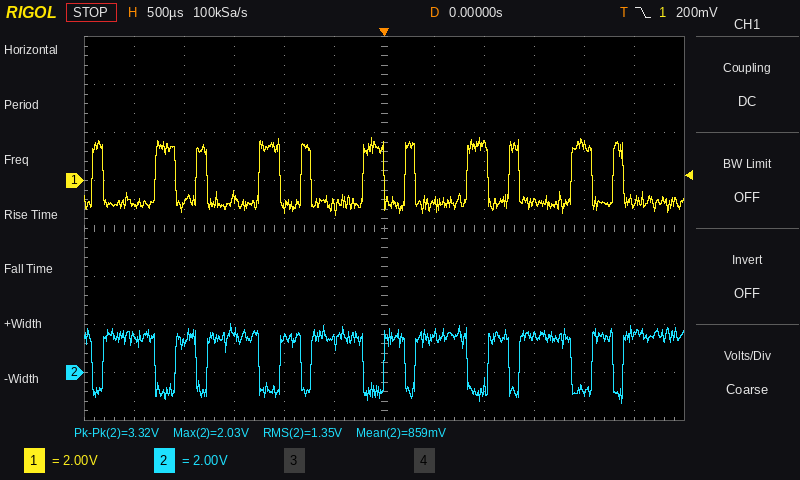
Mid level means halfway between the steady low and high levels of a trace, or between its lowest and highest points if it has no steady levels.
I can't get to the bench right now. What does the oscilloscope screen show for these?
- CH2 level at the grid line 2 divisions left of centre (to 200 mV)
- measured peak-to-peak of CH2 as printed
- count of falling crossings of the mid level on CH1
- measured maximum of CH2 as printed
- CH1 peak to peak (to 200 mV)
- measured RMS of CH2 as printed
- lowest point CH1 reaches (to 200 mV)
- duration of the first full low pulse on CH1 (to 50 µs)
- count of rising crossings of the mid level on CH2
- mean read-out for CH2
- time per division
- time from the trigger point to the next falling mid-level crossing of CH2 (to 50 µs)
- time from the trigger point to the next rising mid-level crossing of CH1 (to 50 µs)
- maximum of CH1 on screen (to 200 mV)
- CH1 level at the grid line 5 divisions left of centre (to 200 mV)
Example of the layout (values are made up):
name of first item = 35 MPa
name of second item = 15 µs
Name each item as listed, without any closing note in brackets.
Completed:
CH2 level at the grid line 2 divisions left of centre = 1.4 V
measured peak-to-peak of CH2 as printed = 3.32 V
count of falling crossings of the mid level on CH1 = 11
measured maximum of CH2 as printed = 2.03 V
CH1 peak to peak = 3.2 V
measured RMS of CH2 as printed = 1.35 V
lowest point CH1 reaches = -1.4 V
duration of the first full low pulse on CH1 = 500 µs
count of rising crossings of the mid level on CH2 = 11
mean read-out for CH2 = 859 mV
time per division = 500 µs
time from the trigger point to the next falling mid-level crossing of CH2 = 200 µs
time from the trigger point to the next rising mid-level crossing of CH1 = 200 µs
maximum of CH1 on screen = 1.8 V
CH1 level at the grid line 5 divisions left of centre = -1.0 V
